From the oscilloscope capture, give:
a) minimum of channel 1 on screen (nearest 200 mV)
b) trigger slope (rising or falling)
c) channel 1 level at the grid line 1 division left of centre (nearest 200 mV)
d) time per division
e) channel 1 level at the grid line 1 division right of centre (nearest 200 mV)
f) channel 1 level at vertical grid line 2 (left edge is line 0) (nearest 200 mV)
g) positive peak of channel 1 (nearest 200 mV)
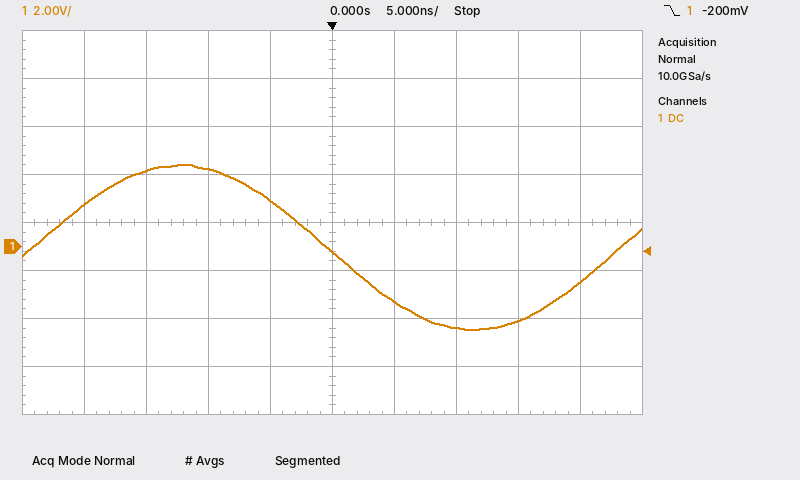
-3.4 V
falling
2.0 V
5 ns
-2.2 V
3.2 V
3.4 V
